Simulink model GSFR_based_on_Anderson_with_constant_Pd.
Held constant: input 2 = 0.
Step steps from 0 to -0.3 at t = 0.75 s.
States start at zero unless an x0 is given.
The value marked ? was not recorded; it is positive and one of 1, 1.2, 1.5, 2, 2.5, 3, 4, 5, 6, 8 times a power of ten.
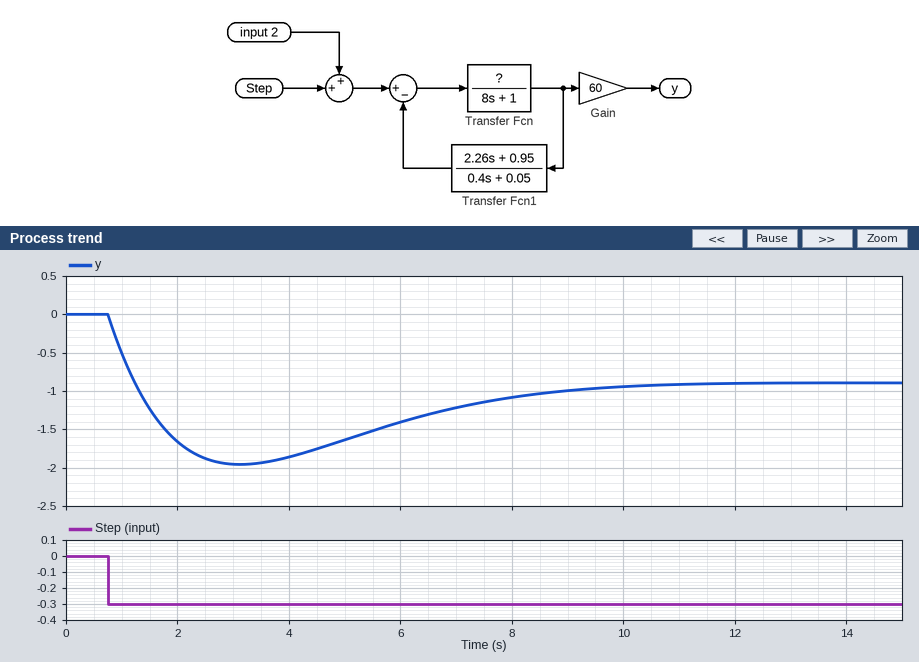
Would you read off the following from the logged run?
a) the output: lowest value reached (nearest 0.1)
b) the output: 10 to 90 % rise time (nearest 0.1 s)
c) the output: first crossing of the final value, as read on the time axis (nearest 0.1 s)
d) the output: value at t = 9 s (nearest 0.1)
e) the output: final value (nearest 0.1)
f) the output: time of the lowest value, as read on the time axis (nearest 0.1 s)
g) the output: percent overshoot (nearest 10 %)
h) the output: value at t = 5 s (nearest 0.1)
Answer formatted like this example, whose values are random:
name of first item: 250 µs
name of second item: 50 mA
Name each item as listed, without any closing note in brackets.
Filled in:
the output: lowest value reached: -2.0
the output: 10 to 90 % rise time: 0.4 s
the output: first crossing of the final value, as read on the time axis: 1.2 s
the output: value at t = 9 s: -1.0
the output: final value: -0.9
the output: time of the lowest value, as read on the time axis: 3.1 s
the output: percent overshoot: 120 %
the output: value at t = 5 s: -1.6
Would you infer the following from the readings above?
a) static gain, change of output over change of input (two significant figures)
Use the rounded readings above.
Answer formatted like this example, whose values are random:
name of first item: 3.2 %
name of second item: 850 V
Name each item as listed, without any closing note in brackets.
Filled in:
static gain, change of output over change of input: 3.0
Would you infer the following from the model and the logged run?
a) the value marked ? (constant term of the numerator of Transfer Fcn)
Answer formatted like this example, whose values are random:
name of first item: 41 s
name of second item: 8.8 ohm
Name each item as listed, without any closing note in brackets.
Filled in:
the value marked ?: 1
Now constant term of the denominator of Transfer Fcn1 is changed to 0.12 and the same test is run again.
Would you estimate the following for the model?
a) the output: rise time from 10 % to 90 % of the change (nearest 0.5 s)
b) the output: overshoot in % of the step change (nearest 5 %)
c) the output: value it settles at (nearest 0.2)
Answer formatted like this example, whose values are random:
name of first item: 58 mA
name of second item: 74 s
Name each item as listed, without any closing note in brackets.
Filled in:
the output: rise time from 10 % to 90 % of the change: 1.5 s
the output: overshoot in % of the step change: 15 %
the output: value it settles at: -2.0
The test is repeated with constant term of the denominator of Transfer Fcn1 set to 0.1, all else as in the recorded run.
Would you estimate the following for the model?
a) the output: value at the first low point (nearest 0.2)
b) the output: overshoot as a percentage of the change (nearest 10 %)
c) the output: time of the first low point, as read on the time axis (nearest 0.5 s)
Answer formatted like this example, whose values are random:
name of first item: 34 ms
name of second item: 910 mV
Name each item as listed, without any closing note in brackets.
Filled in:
the output: value at the first low point: -2.2
the output: overshoot as a percentage of the change: 30 %
the output: time of the first low point, as read on the time axis: 4.0 s
